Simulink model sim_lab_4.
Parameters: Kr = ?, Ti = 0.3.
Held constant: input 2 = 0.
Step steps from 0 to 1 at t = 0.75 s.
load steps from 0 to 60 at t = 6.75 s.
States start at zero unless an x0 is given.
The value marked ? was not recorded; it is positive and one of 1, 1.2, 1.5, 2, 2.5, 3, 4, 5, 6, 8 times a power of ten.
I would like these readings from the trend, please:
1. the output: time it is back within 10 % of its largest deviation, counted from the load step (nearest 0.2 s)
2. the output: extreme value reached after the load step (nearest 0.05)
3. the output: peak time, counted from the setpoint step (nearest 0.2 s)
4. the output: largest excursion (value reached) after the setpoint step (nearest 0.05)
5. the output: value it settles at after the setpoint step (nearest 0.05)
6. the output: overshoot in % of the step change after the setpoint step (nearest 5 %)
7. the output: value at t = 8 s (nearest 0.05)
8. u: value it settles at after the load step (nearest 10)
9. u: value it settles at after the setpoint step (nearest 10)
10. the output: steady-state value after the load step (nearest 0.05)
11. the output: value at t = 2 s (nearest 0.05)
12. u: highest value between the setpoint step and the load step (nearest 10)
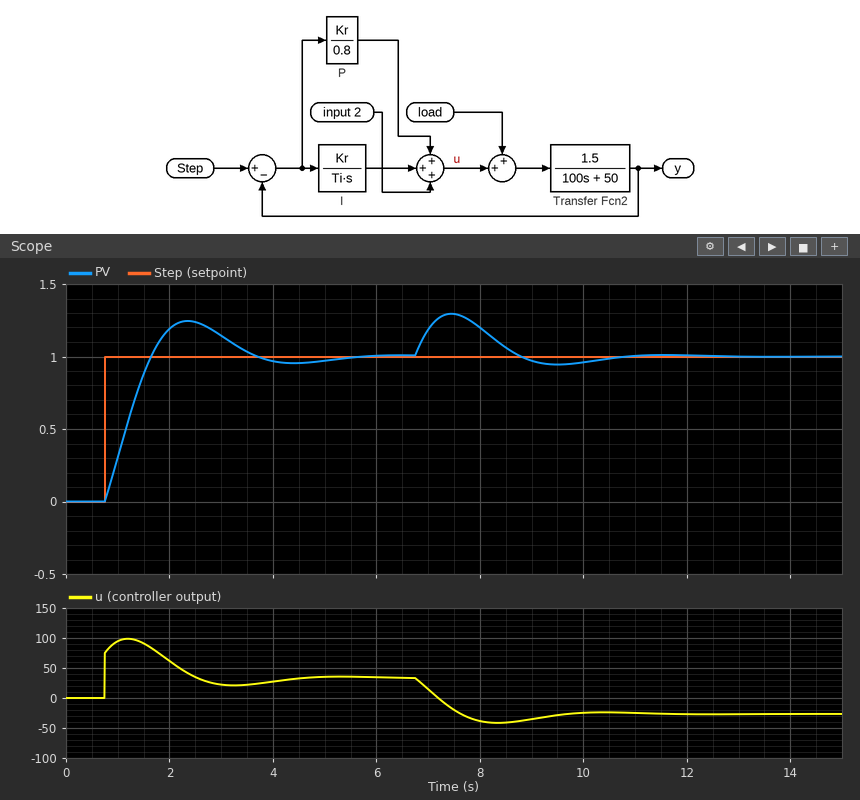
3.4 s
1.30
1.6 s
1.25
1.00
25 %
1.20
-30
30
1.00
1.20
100
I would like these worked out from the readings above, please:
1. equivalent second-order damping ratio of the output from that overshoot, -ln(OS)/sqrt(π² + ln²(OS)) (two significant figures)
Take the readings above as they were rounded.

0.40
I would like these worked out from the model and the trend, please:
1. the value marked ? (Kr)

60
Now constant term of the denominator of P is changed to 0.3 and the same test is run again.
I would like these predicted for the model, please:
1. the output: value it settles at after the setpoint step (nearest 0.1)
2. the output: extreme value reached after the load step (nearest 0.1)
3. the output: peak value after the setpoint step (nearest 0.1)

1.0
1.2
1.1
